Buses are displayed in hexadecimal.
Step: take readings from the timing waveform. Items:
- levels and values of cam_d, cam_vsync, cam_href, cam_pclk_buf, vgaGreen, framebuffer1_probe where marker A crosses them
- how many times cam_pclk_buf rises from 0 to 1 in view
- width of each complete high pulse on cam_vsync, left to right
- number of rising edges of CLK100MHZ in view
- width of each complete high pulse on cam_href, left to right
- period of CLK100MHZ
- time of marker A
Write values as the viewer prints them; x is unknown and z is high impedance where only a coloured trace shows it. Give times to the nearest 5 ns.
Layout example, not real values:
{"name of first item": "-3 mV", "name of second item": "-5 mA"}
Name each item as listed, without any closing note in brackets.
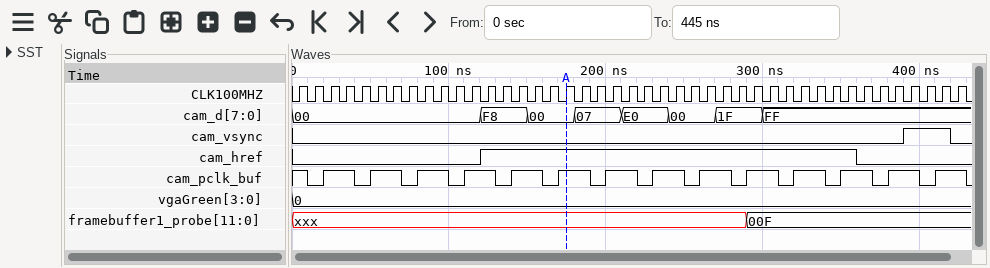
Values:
{"levels and values of cam_d, cam_vsync, cam_href, cam_pclk_buf, vgaGreen, framebuffer1_probe where marker A crosses them": "cam_d=00, cam_vsync=0, cam_href=1, cam_pclk_buf=1, vgaGreen=0, framebuffer1_probe=xxx", "how many times cam_pclk_buf rises from 0 to 1 in view": "14", "width of each complete high pulse on cam_vsync, left to right": "30 ns", "number of rising edges of CLK100MHZ in view": "43", "width of each complete high pulse on cam_href, left to right": "240 ns", "period of CLK100MHZ": "10 ns", "time of marker A": "175 ns"}
